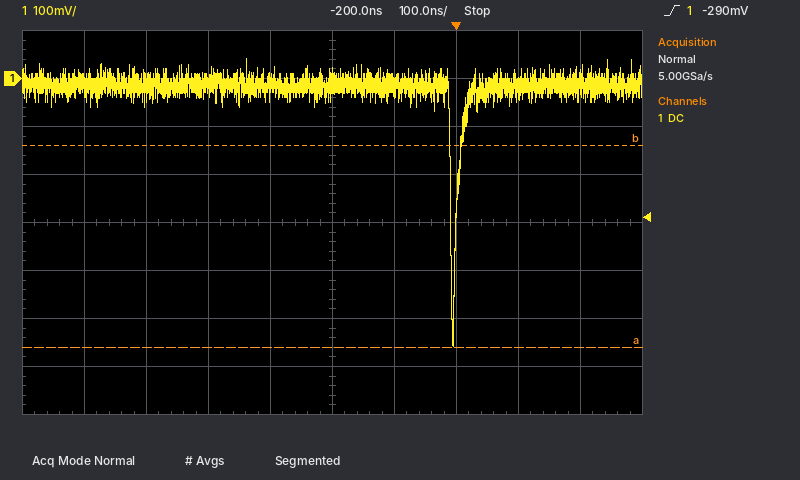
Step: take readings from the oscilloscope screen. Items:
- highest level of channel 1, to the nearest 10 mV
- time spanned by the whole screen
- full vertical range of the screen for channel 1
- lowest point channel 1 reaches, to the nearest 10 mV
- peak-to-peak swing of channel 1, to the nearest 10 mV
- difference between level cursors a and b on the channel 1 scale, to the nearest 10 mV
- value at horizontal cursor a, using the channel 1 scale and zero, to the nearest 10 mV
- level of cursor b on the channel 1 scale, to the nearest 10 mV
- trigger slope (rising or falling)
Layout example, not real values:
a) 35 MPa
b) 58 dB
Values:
a) 40 mV
b) 1 µs
c) 800 mV
d) -560 mV
e) 600 mV
f) 420 mV
g) -560 mV
h) -140 mV
i) rising
